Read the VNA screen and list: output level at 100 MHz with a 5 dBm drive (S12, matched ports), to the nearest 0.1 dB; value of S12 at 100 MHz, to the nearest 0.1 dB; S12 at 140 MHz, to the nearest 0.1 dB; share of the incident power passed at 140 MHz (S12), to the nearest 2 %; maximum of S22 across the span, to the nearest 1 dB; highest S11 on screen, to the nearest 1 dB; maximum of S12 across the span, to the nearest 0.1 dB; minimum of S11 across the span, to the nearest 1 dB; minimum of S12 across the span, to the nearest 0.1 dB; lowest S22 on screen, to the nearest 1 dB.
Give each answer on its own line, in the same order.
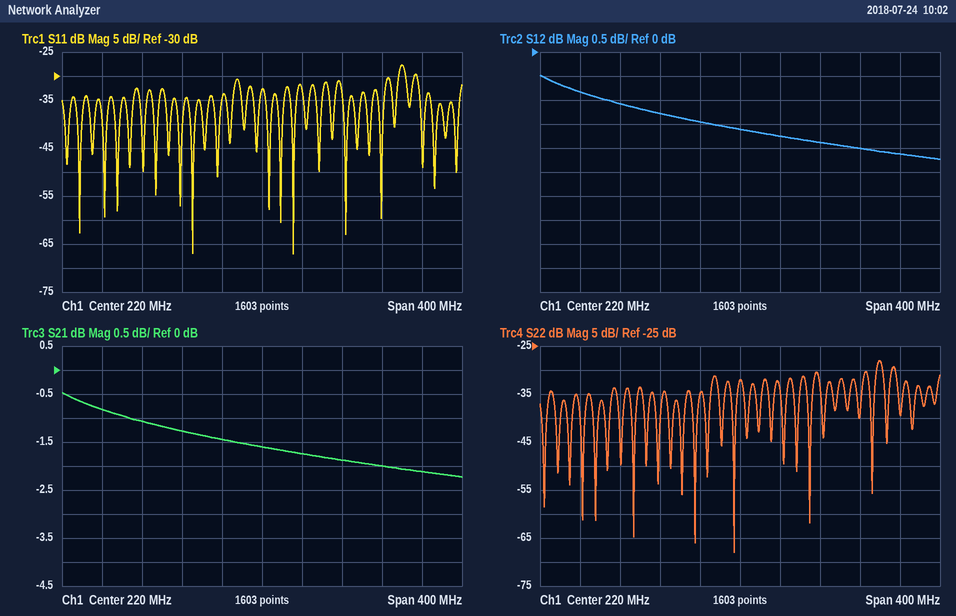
3.9 dBm
-1.1 dB
-1.3 dB
74 %
-28 dB
-28 dB
-0.5 dB
-67 dB
-2.2 dB
-68 dB
